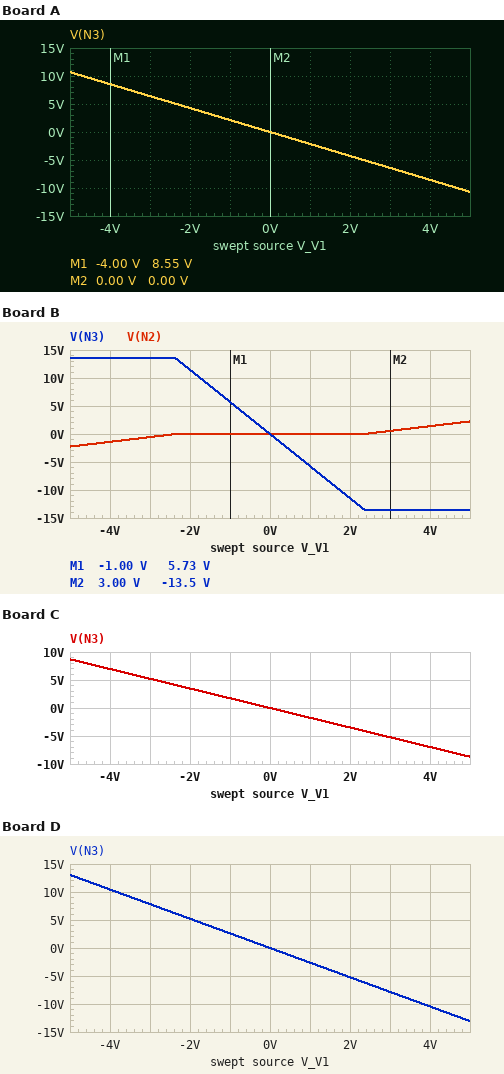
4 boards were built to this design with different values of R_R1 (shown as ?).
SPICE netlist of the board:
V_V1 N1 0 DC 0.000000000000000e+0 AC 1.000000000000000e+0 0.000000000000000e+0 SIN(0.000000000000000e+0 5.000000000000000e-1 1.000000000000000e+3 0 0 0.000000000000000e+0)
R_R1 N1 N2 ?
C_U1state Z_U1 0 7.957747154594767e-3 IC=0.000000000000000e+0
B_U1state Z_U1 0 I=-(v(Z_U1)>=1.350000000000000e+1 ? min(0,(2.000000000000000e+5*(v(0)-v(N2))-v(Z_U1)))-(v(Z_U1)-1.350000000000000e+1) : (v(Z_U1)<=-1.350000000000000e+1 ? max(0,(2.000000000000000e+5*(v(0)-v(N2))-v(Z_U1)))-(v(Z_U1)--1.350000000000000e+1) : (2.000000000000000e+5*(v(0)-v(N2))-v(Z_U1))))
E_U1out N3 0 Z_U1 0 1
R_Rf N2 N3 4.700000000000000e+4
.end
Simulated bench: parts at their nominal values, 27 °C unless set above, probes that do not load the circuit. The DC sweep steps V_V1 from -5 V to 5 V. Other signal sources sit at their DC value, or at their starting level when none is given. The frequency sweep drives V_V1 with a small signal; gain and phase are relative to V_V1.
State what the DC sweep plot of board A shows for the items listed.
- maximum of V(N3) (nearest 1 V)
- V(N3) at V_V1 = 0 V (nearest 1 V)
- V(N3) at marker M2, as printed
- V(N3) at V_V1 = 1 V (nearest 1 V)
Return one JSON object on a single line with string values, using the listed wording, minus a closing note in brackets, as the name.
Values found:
{"maximum of V(N3)": "11 V", "V(N3) at V_V1 = 0 V": "0 V", "V(N3) at marker M2, as printed": "0.00 V", "V(N3) at V_V1 = 1 V": "-2 V"}
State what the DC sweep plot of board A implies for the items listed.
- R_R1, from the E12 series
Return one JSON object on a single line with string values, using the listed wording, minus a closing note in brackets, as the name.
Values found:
{"R_R1, from the E12 series": "22 kΩ"}
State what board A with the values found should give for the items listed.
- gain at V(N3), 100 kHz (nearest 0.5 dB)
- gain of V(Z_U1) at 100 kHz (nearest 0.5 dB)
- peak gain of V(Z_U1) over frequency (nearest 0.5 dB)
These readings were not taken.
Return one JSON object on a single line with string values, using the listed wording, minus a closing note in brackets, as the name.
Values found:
{"gain at V(N3), 100 kHz": "6.5 dB", "gain of V(Z_U1) at 100 kHz": "6.5 dB", "peak gain of V(Z_U1) over frequency": "6.5 dB"}
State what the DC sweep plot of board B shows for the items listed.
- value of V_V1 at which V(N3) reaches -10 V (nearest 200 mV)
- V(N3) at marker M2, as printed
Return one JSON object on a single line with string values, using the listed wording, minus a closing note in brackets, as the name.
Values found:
{"value of V_V1 at which V(N3) reaches -10 V": "1.8 V", "V(N3) at marker M2, as printed": "-13.5 V"}
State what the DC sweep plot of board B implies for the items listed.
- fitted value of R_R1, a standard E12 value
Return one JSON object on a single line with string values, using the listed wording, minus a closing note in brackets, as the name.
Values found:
{"fitted value of R_R1, a standard E12 value": "8.2 kΩ"}
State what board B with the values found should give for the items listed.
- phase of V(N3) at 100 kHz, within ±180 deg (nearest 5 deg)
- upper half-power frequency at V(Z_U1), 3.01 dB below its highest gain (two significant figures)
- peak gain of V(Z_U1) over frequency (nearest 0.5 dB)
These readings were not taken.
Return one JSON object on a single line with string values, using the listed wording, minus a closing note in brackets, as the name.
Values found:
{"phase of V(N3) at 100 kHz, within ±180 deg": "170 deg", "upper half-power frequency at V(Z_U1), 3.01 dB below its highest gain": "590 kHz", "peak gain of V(Z_U1) over frequency": "15.0 dB"}
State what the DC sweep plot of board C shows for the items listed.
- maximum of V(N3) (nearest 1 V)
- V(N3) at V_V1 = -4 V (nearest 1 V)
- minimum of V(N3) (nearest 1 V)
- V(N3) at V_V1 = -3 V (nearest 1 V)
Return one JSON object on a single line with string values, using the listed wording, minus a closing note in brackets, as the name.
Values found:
{"maximum of V(N3)": "9 V", "V(N3) at V_V1 = -4 V": "7 V", "minimum of V(N3)": "-9 V", "V(N3) at V_V1 = -3 V": "5 V"}
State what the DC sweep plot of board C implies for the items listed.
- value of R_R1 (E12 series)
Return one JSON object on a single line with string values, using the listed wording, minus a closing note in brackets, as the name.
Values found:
{"value of R_R1": "27 kΩ"}
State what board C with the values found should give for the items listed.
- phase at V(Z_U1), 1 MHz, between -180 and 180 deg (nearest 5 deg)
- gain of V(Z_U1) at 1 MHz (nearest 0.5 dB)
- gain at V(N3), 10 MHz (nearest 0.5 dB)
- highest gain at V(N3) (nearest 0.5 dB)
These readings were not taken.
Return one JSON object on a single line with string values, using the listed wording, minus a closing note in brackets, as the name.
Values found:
{"phase at V(Z_U1), 1 MHz, between -180 and 180 deg": "145 deg", "gain of V(Z_U1) at 1 MHz": "3.0 dB", "gain at V(N3), 10 MHz": "-12.0 dB", "highest gain at V(N3)": "5.0 dB"}
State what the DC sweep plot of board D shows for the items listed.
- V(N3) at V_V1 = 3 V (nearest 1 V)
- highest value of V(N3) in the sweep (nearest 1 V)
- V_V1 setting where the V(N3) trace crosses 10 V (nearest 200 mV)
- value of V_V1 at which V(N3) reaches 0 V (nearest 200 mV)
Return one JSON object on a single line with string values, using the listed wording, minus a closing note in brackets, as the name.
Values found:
{"V(N3) at V_V1 = 3 V": "-8 V", "highest value of V(N3) in the sweep": "13 V", "V_V1 setting where the V(N3) trace crosses 10 V": "-3.8 V", "value of V_V1 at which V(N3) reaches 0 V": "0 V"}
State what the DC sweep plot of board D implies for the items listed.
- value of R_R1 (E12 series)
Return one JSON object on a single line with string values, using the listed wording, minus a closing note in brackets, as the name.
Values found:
{"value of R_R1": "18 kΩ"}
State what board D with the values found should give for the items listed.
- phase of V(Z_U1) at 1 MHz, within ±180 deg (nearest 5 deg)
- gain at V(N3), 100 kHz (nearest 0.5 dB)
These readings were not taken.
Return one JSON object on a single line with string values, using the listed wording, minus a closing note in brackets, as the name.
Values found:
{"phase of V(Z_U1) at 1 MHz, within ±180 deg": "140 deg", "gain at V(N3), 100 kHz": "8.5 dB"}
